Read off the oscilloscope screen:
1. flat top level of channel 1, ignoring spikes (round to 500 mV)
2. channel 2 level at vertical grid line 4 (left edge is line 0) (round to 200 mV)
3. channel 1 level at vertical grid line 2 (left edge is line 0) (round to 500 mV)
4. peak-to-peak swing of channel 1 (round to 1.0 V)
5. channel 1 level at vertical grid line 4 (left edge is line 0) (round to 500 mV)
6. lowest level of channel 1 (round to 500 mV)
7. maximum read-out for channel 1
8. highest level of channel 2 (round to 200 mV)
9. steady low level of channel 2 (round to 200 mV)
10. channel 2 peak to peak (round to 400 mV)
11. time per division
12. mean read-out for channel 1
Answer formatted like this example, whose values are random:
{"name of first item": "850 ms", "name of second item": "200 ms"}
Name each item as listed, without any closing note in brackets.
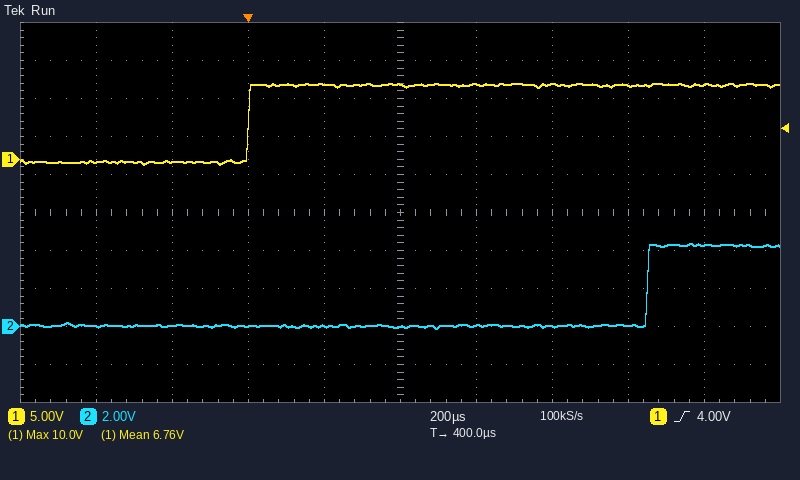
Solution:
{"flat top level of channel 1, ignoring spikes": "10.0 V", "channel 2 level at vertical grid line 4 (left edge is line 0)": "0.0 V", "channel 1 level at vertical grid line 2 (left edge is line 0)": "-500 mV", "peak-to-peak swing of channel 1": "11.0 V", "channel 1 level at vertical grid line 4 (left edge is line 0)": "10.0 V", "lowest level of channel 1": "-500 mV", "maximum read-out for channel 1": "10.0 V", "highest level of channel 2": "4.4 V", "steady low level of channel 2": "0.0 V", "channel 2 peak to peak": "4.4 V", "time per division": "200 µs", "mean read-out for channel 1": "6.76 V"}
